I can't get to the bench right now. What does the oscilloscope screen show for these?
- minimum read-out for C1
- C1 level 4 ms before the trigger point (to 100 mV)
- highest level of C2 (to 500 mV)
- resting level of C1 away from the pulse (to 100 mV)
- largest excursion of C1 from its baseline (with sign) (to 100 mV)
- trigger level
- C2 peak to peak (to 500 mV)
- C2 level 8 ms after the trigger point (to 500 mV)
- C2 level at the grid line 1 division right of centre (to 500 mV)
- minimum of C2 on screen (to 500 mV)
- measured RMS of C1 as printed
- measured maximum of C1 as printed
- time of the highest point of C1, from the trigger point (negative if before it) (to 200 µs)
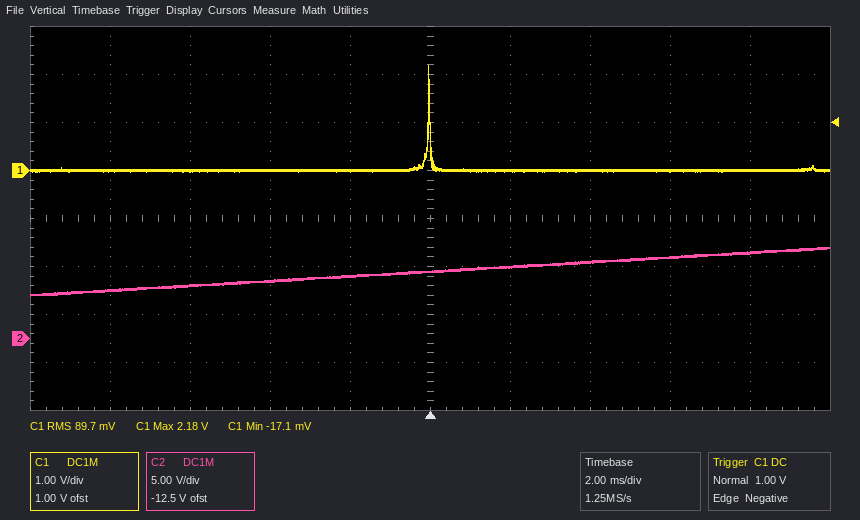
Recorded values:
-17.1 mV
0.0 V
9.5 V
0.0 V
+2.2 V
1.00 V
5.0 V
9.0 V
7.5 V
4.5 V
89.7 mV
2.18 V
0.0 ms
